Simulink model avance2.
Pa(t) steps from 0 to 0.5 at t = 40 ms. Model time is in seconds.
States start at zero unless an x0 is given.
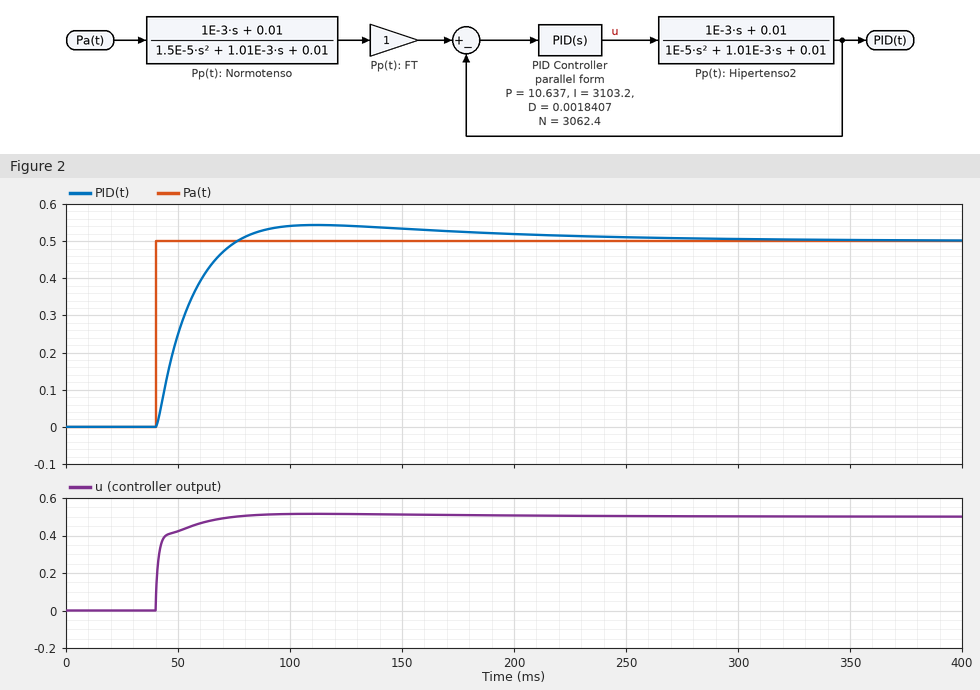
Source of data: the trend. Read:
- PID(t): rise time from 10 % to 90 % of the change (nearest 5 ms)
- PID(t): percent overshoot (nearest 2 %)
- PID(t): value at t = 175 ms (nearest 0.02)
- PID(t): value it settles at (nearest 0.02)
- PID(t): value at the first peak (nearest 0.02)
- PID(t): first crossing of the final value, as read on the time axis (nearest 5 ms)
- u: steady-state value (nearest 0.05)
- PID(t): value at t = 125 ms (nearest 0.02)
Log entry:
25 ms
8 %
0.52
0.50
0.54
75 ms
0.50
0.54
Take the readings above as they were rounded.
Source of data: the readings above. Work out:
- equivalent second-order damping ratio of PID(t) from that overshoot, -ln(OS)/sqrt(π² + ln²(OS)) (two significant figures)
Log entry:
0.63
